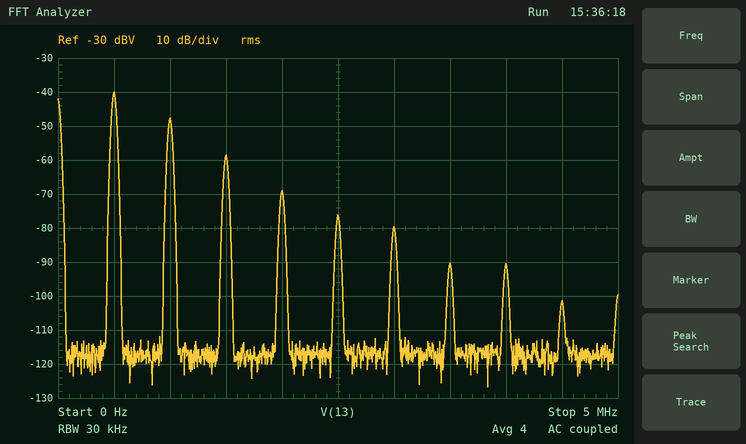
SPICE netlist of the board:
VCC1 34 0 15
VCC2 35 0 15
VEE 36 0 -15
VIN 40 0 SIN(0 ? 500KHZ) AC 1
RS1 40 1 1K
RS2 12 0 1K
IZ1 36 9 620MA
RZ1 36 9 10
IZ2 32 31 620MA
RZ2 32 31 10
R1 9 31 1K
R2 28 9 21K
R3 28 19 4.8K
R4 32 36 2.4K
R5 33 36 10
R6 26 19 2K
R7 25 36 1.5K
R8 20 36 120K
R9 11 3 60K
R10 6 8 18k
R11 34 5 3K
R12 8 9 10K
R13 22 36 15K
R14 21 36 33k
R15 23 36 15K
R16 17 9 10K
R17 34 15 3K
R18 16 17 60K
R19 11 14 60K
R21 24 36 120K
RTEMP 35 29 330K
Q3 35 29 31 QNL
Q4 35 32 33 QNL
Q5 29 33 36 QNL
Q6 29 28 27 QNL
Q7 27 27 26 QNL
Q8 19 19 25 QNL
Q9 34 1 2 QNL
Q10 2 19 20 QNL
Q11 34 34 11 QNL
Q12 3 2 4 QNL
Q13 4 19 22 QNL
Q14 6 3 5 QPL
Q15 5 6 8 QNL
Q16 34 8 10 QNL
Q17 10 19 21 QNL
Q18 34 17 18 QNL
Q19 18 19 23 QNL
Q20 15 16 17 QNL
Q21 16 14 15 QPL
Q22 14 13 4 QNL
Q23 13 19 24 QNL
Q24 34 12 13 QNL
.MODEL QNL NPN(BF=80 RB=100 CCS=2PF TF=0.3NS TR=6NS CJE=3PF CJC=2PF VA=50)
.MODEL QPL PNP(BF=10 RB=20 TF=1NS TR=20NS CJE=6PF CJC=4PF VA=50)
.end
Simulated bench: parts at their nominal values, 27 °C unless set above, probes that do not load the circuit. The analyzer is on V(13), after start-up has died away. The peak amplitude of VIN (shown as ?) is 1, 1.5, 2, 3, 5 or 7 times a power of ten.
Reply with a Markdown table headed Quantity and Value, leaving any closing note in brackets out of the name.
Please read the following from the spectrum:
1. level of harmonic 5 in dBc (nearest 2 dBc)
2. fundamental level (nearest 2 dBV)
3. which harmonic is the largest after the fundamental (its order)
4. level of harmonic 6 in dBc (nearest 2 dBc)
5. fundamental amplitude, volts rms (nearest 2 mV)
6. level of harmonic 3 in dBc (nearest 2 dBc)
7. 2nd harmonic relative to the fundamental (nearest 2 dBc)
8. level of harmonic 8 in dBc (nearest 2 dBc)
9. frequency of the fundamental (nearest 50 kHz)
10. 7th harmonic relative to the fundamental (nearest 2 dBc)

| Quantity | Value |
|---|---|
| level of harmonic 5 in dBc | -36 dBc |
| fundamental level | -40 dBV |
| which harmonic is the largest after the fundamental | 2 |
| level of harmonic 6 in dBc | -40 dBc |
| fundamental amplitude, volts rms | 10 mV |
| level of harmonic 3 in dBc | -18 dBc |
| 2nd harmonic relative to the fundamental | -8 dBc |
| level of harmonic 8 in dBc | -50 dBc |
| frequency of the fundamental | 500 kHz |
| 7th harmonic relative to the fundamental | -50 dBc |
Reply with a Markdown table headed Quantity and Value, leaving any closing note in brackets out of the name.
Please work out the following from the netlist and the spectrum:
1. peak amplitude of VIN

| Quantity | Value |
|---|---|
| peak amplitude of VIN | 150 mV |
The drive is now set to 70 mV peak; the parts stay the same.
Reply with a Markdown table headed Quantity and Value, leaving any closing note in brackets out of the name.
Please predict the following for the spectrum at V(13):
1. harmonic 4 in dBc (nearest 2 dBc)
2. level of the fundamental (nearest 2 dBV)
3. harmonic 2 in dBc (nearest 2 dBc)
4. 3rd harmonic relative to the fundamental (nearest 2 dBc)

| Quantity | Value |
|---|---|
| harmonic 4 in dBc | -46 dBc |
| level of the fundamental | -46 dBV |
| harmonic 2 in dBc | -14 dBc |
| 3rd harmonic relative to the fundamental | -26 dBc |
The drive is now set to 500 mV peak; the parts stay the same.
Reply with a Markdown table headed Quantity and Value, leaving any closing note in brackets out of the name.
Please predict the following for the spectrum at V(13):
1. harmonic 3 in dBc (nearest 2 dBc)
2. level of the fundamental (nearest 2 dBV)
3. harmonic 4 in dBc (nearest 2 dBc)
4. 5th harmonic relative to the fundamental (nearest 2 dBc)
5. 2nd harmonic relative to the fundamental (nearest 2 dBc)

| Quantity | Value |
|---|---|
| harmonic 3 in dBc | -16 dBc |
| level of the fundamental | -30 dBV |
| harmonic 4 in dBc | -26 dBc |
| 5th harmonic relative to the fundamental | -26 dBc |
| 2nd harmonic relative to the fundamental | -4 dBc |
